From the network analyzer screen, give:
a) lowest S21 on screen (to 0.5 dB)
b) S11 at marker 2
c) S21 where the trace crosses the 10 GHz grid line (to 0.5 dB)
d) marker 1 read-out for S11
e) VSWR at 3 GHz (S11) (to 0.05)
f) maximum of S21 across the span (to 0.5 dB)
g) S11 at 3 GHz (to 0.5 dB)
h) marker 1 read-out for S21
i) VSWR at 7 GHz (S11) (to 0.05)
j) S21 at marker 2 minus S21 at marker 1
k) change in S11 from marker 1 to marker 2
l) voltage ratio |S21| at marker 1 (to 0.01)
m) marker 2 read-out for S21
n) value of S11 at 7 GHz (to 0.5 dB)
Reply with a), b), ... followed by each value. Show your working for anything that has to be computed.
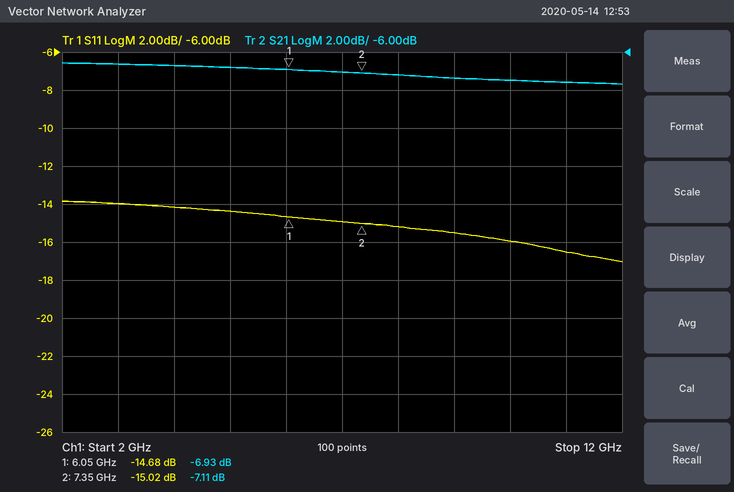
a) -7.5 dB
b) -15.02 dB
c) -7.5 dB
d) -14.68 dB
e) |Γ| = 10^(-14/20) = 0.1995; VSWR = (1 + 0.1995)/(1 − 0.1995) ≈ 1.50
f) -6.5 dB
g) -14.0 dB
h) -6.93 dB
i) |Γ| = 10^(-15/20) = 0.1778; VSWR = (1 + 0.1778)/(1 − 0.1778) ≈ 1.43, so 1.45 to the nearest 0.05
j) -7.11 − (-6.93) = -0.18 dB
k) -15.02 − (-14.68) = -0.34 dB
l) 10^(-6.93/20) ≈ 0.45
m) -7.11 dB
n) -15.0 dB
